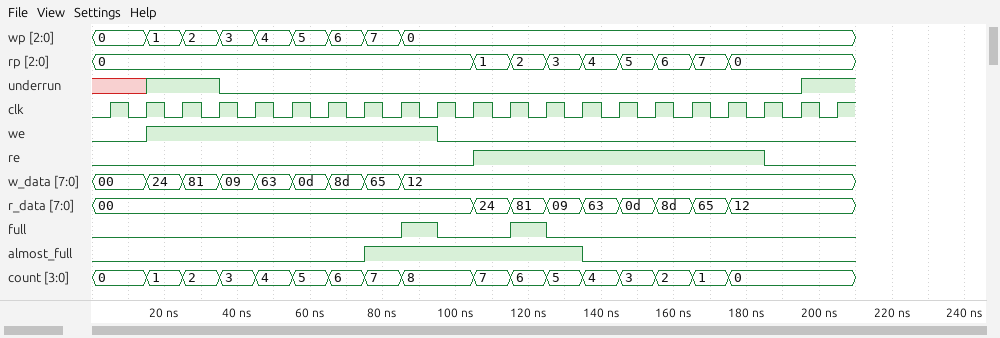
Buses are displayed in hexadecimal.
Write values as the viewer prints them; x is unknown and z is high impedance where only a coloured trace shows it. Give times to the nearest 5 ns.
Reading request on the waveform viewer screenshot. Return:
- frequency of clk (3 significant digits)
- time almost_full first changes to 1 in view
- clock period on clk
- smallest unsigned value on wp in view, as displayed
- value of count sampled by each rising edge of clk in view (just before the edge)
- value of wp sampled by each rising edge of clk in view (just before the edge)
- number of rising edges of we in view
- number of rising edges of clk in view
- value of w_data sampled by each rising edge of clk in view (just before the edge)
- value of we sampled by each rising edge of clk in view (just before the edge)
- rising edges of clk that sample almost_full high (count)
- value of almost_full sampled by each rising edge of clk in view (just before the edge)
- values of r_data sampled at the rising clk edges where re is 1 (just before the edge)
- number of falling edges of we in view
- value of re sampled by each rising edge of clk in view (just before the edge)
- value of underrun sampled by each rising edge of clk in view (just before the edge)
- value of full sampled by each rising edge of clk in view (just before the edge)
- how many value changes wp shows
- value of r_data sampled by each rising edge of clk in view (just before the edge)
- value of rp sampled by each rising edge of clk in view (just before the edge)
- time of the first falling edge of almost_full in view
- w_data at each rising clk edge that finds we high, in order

100 MHz
75 ns
10 ns
0
0, 0, 1, 2, 3, 4, 5, 6, 7, 8, 8, 7, 6, 5, 4, 3, 2, 1, 0, 0, 0
0, 0, 1, 2, 3, 4, 5, 6, 7, 0, 0, 0, 0, 0, 0, 0, 0, 0, 0, 0, 0
1
21
00, 00, 24, 81, 09, 63, 0d, 8d, 65, 12, 12, 12, 12, 12, 12, 12, 12, 12, 12, 12, 12
0 0 1 1 1 1 1 1 1 1 0 0 0 0 0 0 0 0 0 0 0
6
0 0 0 0 0 0 0 0 1 1 1 1 1 1 0 0 0 0 0 0 0
24, 81, 09, 63, 0d, 8d, 65, 12
1
0 0 0 0 0 0 0 0 0 0 0 1 1 1 1 1 1 1 1 0 0
x x 1 1 0 0 0 0 0 0 0 0 0 0 0 0 0 0 0 0 1
0 0 0 0 0 0 0 0 0 1 0 0 1 0 0 0 0 0 0 0 0
8
00, 00, 00, 00, 00, 00, 00, 00, 00, 00, 00, 24, 81, 09, 63, 0d, 8d, 65, 12, 12, 12
0, 0, 0, 0, 0, 0, 0, 0, 0, 0, 0, 1, 2, 3, 4, 5, 6, 7, 0, 0, 0
135 ns
24, 81, 09, 63, 0d, 8d, 65, 12
